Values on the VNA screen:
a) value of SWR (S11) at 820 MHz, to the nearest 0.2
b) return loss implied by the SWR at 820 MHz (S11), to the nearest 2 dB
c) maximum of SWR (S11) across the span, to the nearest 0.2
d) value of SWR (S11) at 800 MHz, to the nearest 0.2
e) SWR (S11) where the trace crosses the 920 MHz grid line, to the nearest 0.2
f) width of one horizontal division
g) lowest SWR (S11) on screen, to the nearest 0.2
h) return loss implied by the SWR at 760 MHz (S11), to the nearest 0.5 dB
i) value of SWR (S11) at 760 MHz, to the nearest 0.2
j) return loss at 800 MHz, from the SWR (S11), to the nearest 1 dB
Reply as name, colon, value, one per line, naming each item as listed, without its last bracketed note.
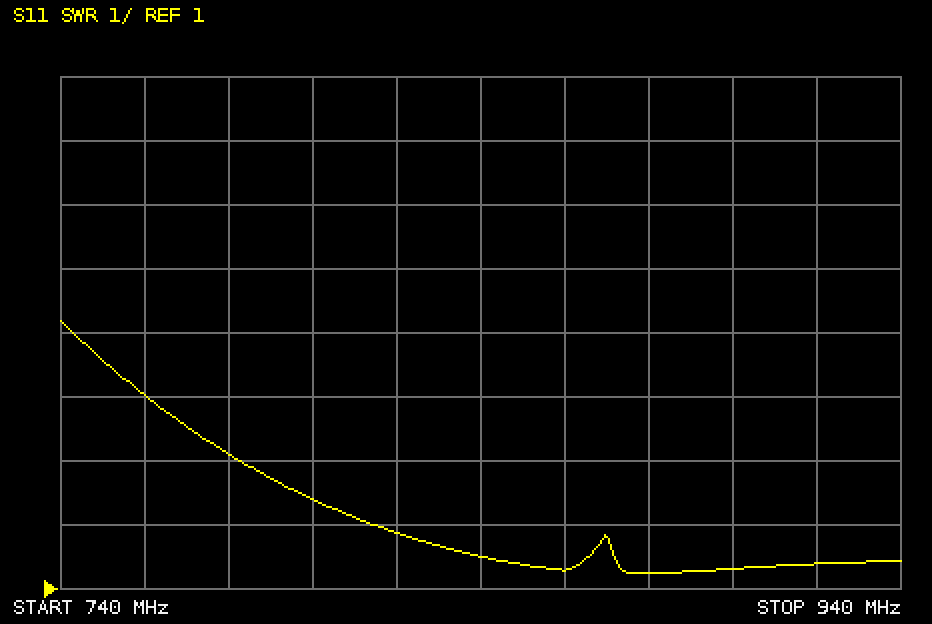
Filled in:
value of SWR (S11) at 820 MHz, to the nearest 0.2: 1.8
return loss implied by the SWR at 820 MHz (S11), to the nearest 2 dB: 10 dB
maximum of SWR (S11) across the span, to the nearest 0.2: 5.2
value of SWR (S11) at 800 MHz, to the nearest 0.2: 2.4
SWR (S11) where the trace crosses the 920 MHz grid line, to the nearest 0.2: 1.4
width of one horizontal division: 20 MHz
lowest SWR (S11) on screen, to the nearest 0.2: 1.2
return loss implied by the SWR at 760 MHz (S11), to the nearest 0.5 dB: 4.5 dB
value of SWR (S11) at 760 MHz, to the nearest 0.2: 4.0
return loss at 800 MHz, from the SWR (S11), to the nearest 1 dB: 8 dB
